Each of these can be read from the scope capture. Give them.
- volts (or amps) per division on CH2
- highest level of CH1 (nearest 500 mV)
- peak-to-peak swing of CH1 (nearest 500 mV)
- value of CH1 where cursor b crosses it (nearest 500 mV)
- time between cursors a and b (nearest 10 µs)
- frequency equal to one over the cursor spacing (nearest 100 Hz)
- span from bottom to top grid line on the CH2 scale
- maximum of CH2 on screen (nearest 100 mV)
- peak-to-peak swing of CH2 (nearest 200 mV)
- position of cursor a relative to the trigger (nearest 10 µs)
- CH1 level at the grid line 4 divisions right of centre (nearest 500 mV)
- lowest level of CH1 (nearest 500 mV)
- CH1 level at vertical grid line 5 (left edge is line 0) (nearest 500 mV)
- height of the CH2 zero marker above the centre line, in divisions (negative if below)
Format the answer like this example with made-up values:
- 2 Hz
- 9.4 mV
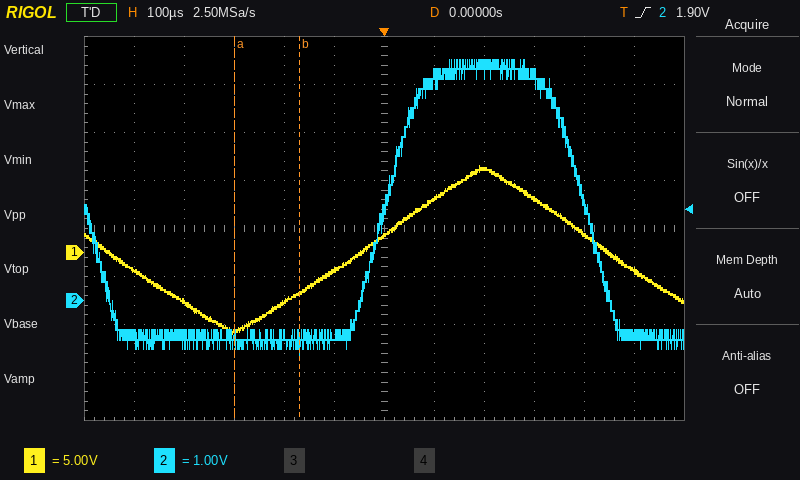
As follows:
- 1 V
- 9.0 V
- 17.5 V
- -4.0 V
- 130 µs
- 7.7 kHz
- 8 V
- 5.0 V
- 6.2 V
- -300 µs
- 2.0 V
- -8.5 V
- -2.0 V
- -1.5 div
